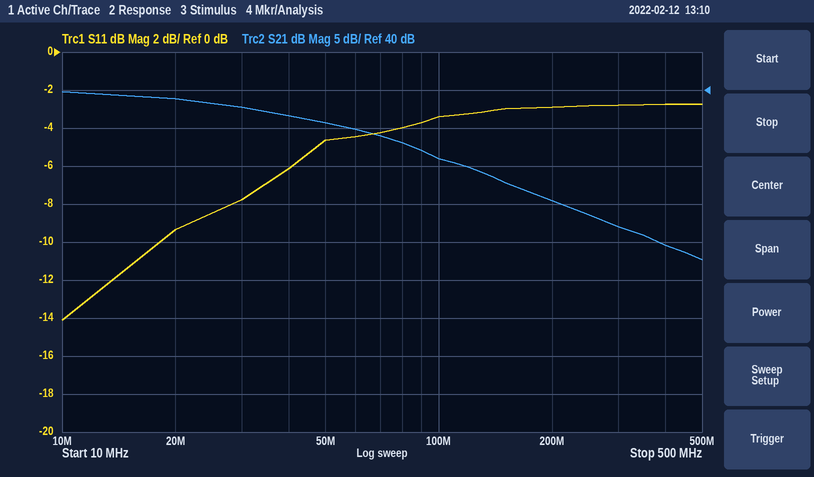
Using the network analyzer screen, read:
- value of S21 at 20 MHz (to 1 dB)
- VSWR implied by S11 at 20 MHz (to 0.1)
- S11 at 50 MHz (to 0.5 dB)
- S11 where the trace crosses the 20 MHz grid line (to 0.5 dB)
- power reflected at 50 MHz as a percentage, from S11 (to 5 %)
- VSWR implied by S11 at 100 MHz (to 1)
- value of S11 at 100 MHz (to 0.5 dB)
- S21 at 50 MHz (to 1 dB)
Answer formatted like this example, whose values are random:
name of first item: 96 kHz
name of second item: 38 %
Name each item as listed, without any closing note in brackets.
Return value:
value of S21 at 20 MHz: 39 dB
VSWR implied by S11 at 20 MHz: 2.0
S11 at 50 MHz: -4.5 dB
S11 where the trace crosses the 20 MHz grid line: -9.5 dB
power reflected at 50 MHz as a percentage, from S11: 35 %
VSWR implied by S11 at 100 MHz: 5
value of S11 at 100 MHz: -3.5 dB
S21 at 50 MHz: 36 dB
